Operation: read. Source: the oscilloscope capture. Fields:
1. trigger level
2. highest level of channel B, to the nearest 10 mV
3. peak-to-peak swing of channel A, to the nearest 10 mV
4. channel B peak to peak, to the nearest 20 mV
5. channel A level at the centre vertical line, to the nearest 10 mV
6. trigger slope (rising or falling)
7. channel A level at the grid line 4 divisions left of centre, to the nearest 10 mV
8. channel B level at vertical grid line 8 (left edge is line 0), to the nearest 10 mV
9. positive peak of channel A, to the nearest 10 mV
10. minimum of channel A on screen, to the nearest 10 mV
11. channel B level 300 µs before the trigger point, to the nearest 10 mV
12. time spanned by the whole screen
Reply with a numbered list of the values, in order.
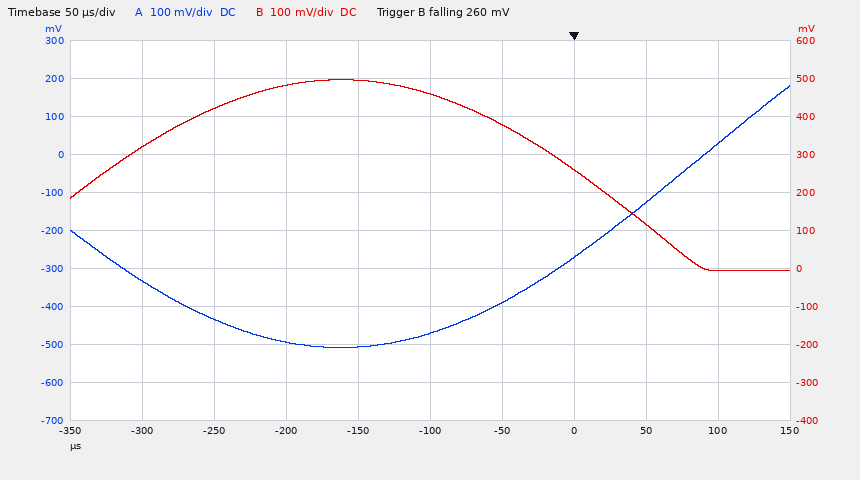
1. 260 mV
2. 500 mV
3. 690 mV
4. 500 mV
5. -470 mV
6. falling
7. -330 mV
8. 120 mV
9. 180 mV
10. -510 mV
11. 320 mV
12. 500 µs
